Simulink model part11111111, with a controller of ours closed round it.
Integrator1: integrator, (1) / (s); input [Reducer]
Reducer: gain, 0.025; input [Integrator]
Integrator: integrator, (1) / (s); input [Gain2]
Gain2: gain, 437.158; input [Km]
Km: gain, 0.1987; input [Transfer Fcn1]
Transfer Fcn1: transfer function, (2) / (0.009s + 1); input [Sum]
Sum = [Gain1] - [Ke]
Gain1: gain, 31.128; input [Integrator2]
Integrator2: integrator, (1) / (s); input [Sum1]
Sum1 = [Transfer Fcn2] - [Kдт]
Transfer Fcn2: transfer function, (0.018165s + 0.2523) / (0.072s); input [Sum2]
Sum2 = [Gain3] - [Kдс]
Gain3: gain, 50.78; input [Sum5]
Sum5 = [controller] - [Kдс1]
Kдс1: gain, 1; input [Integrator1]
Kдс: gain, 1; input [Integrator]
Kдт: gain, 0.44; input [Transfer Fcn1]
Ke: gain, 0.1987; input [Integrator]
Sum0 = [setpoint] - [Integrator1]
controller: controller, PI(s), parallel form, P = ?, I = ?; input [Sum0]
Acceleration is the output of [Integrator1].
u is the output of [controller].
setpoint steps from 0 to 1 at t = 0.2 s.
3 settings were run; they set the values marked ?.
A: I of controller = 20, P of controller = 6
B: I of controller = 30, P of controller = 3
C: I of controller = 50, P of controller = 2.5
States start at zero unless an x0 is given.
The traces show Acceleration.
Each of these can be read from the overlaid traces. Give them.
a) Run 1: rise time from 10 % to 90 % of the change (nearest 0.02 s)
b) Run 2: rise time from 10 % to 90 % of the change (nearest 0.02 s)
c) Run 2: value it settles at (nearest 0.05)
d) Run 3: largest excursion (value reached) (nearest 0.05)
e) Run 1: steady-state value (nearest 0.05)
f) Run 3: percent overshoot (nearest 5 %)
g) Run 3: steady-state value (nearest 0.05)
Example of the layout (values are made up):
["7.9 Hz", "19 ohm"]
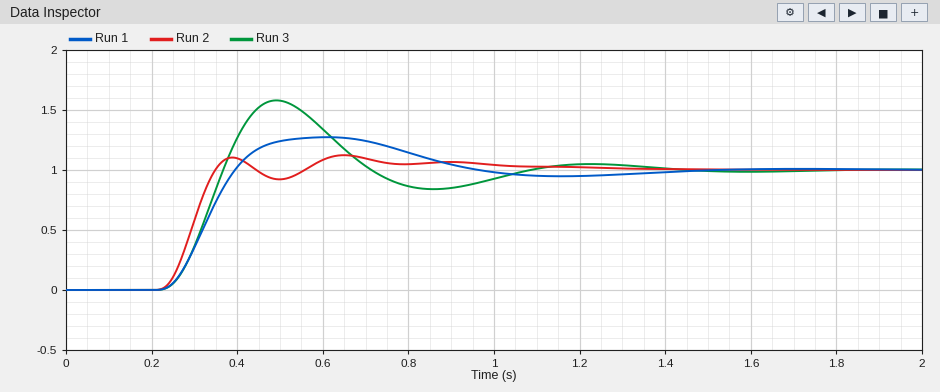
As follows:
["0.12 s", "0.08 s", "1.00", "1.60", "1.00", "60 %", "1.00"]
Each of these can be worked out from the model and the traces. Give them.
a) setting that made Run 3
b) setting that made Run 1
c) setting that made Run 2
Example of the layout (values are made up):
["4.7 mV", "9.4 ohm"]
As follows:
["C", "B", "A"]
